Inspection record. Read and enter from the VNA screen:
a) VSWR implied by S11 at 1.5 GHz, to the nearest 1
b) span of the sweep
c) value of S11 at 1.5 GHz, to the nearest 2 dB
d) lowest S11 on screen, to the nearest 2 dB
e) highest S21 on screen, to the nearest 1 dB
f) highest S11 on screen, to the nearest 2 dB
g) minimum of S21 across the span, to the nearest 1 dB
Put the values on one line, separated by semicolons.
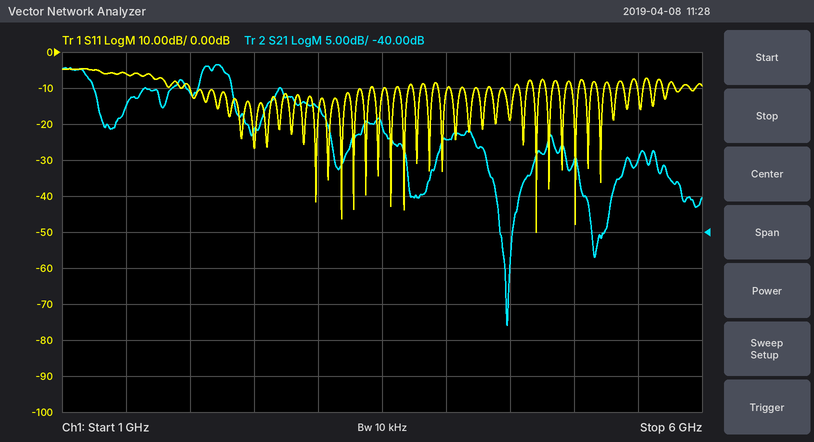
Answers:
3; 5 GHz; -6 dB; -50 dB; -17 dB; -4 dB; -53 dB
